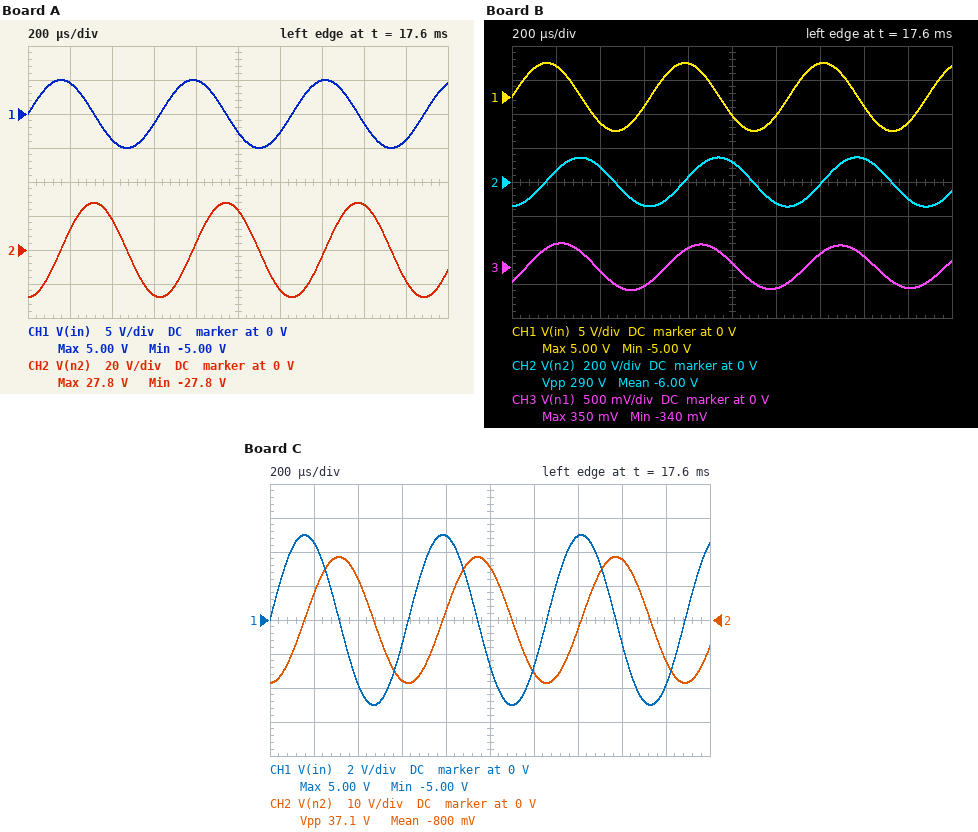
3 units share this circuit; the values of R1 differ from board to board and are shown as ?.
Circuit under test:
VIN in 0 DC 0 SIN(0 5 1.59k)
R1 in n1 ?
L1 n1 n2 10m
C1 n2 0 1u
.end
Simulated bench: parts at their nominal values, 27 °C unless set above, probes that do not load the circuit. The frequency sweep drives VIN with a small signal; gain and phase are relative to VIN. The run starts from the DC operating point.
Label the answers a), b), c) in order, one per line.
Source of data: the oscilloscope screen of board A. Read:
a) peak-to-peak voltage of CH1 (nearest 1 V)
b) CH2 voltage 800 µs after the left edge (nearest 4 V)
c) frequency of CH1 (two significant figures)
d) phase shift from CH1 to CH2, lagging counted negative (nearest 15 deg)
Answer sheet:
a) 10 V
b) 4 V
c) 1.6 kHz
d) -90 deg
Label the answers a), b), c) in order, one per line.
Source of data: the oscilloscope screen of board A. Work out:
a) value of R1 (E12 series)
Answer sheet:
a) 18 Ω
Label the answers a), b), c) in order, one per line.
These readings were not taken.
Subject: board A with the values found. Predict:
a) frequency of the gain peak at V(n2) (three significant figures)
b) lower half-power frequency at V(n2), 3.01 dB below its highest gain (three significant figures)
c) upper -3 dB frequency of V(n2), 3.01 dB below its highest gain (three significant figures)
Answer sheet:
a) 1.58 kHz
b) 1.43 kHz
c) 1.72 kHz
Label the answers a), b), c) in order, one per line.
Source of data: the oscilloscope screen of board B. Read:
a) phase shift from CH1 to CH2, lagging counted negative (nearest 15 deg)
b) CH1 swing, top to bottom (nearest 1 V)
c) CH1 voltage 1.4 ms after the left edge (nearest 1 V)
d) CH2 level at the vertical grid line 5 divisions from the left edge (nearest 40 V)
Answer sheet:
a) -90 deg
b) 10 V
c) 5 V
d) 120 V
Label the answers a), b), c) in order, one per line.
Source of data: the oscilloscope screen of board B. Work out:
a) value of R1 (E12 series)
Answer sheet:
a) 3.3 Ω
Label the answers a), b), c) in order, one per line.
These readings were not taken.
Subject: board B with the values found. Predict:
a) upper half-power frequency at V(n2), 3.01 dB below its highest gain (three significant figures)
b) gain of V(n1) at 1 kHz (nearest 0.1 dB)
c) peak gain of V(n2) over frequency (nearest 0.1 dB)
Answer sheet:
a) 1.62 kHz
b) 0 dB
c) 29.6 dB
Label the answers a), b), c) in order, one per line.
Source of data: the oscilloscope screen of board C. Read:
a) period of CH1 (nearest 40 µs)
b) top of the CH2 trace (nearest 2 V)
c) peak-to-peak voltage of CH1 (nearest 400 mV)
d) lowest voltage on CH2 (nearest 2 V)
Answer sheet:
a) 640 µs
b) 18 V
c) 10.0 V
d) -18 V
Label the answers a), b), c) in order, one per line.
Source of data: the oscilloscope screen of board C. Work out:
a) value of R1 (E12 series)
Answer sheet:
a) 27 Ω
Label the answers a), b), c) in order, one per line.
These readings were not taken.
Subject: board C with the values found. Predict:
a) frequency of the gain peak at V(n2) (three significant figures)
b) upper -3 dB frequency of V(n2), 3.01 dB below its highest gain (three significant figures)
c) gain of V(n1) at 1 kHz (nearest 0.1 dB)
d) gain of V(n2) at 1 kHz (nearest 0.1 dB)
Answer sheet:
a) 1.56 kHz
b) 1.77 kHz
c) -0.3 dB
d) 4.0 dB
